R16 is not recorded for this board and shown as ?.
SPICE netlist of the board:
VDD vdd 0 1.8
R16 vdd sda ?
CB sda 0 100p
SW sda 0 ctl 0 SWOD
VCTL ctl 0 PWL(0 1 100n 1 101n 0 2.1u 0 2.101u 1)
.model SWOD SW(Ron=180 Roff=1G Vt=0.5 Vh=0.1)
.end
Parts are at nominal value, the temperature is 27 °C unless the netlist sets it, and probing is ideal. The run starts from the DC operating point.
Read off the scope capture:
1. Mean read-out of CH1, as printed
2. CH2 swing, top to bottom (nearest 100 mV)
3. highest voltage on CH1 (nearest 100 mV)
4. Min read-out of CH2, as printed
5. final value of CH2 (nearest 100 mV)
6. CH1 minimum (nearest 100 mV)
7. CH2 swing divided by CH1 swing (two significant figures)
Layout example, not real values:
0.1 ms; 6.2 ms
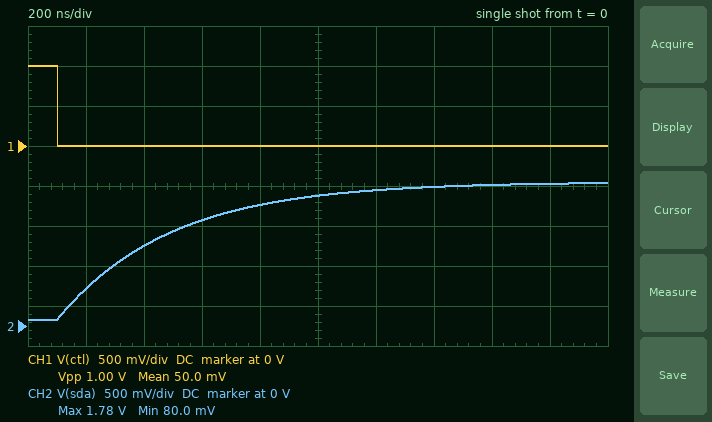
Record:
50.0 mV; 1.7 V; 1.0 V; 80.0 mV; 1.8 V; 0 V; 1.7
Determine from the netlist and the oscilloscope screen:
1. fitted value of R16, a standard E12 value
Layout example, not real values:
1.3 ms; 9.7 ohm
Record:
3.9 kΩ
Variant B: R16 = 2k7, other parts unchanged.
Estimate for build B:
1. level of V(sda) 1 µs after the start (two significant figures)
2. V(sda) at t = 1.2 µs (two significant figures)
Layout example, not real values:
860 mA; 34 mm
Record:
1.7 V; 1.8 V
